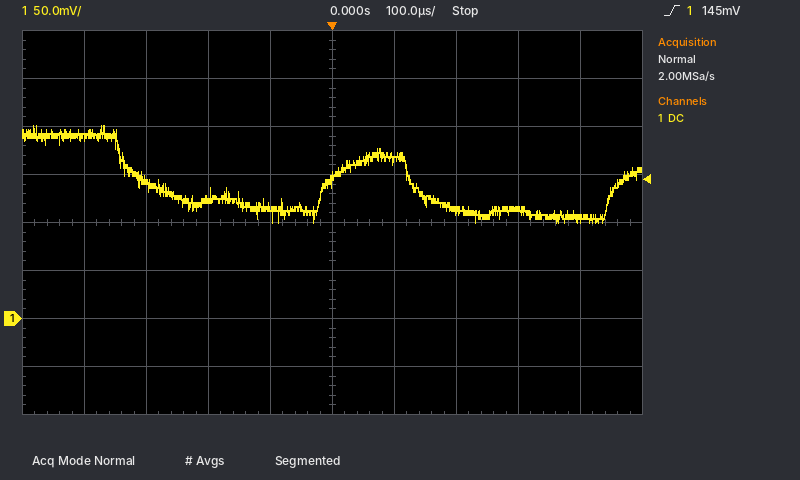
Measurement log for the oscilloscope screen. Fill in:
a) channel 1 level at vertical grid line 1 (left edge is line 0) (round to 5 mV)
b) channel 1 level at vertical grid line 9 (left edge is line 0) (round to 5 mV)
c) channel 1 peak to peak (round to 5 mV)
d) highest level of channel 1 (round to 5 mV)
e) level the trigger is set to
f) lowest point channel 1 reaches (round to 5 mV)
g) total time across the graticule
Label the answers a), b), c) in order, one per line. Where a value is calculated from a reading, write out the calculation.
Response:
a) 190 mV
b) 105 mV
c) 200 mV − (100 mV) = 100 mV
d) 200 mV
e) 145 mV
f) 100 mV
g) 1 ms
